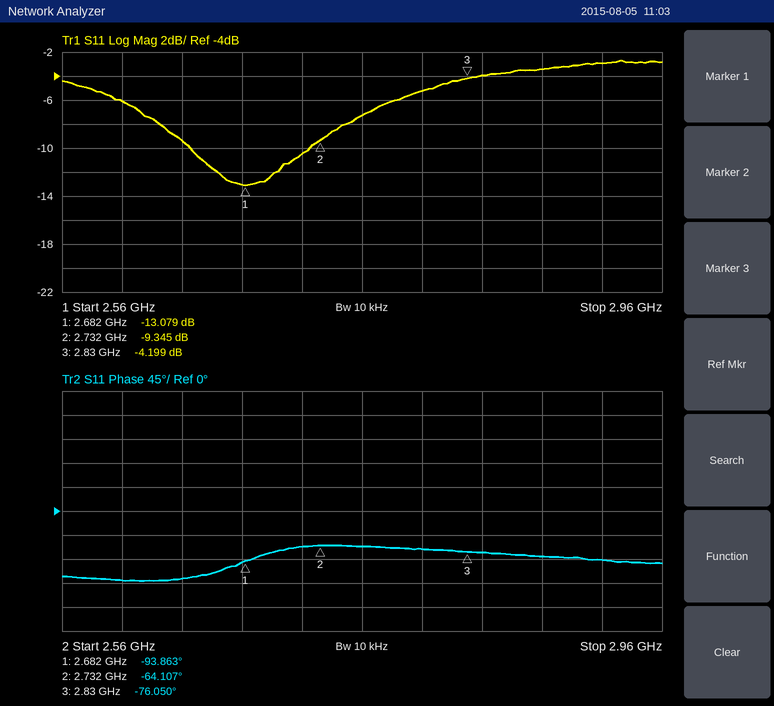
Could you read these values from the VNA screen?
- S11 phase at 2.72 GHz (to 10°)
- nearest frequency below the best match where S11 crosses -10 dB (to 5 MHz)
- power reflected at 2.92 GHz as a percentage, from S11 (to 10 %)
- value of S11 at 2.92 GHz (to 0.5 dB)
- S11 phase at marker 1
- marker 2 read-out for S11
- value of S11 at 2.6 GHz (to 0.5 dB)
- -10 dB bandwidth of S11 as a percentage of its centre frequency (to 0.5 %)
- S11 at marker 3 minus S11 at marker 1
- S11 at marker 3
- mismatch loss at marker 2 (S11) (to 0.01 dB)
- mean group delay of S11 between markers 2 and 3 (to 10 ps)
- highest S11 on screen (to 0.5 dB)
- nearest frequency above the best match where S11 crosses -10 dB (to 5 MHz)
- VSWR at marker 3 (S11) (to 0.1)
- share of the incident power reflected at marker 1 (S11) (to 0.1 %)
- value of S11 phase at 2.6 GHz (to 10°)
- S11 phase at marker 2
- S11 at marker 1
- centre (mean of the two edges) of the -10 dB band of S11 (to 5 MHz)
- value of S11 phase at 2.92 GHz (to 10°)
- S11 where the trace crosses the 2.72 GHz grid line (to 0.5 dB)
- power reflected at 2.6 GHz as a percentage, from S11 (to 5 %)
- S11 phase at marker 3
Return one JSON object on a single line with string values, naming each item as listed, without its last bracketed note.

{"S11 phase at 2.72 GHz": "-70°", "nearest frequency below the best match where S11 crosses -10 dB": "2.645 GHz", "power reflected at 2.92 GHz as a percentage, from S11": "50 %", "value of S11 at 2.92 GHz": "-3.0 dB", "S11 phase at marker 1": "-93.863°", "marker 2 read-out for S11": "-9.345 dB", "value of S11 at 2.6 GHz": "-6.0 dB", "-10 dB bandwidth of S11 as a percentage of its centre frequency": "3.0 %", "S11 at marker 3 minus S11 at marker 1": "8.880 dB", "S11 at marker 3": "-4.199 dB", "mismatch loss at marker 2 (S11)": "0.54 dB", "mean group delay of S11 between markers 2 and 3": "340 ps", "highest S11 on screen": "-2.5 dB", "nearest frequency above the best match where S11 crosses -10 dB": "2.725 GHz", "VSWR at marker 3 (S11)": "4.2", "share of the incident power reflected at marker 1 (S11)": "4.9 %", "value of S11 phase at 2.6 GHz": "-130°", "S11 phase at marker 2": "-64.107°", "S11 at marker 1": "-13.079 dB", "centre (mean of the two edges) of the -10 dB band of S11": "2.685 GHz", "value of S11 phase at 2.92 GHz": "-90°", "S11 where the trace crosses the 2.72 GHz grid line": "-10.5 dB", "power reflected at 2.6 GHz as a percentage, from S11": "25 %", "S11 phase at marker 3": "-76.050°"}
